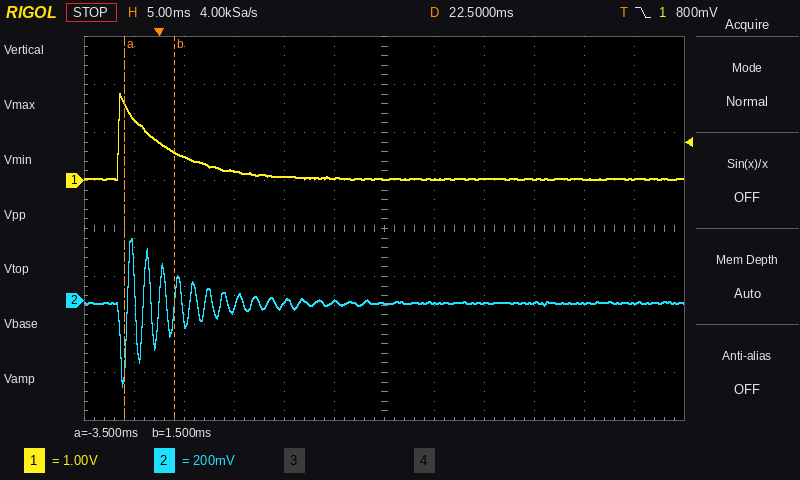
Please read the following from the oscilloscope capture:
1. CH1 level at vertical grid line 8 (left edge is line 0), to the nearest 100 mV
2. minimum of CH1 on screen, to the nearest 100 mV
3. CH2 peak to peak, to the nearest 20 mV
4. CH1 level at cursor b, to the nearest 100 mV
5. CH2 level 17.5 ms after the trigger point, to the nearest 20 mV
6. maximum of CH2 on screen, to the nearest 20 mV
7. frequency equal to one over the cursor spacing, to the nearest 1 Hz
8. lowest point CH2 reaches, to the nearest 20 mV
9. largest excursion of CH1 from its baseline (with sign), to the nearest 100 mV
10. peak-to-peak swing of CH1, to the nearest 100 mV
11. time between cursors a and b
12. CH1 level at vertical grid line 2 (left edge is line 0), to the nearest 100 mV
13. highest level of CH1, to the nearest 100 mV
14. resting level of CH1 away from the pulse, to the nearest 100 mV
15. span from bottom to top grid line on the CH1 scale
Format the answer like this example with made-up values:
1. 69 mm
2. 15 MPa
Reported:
1. 0.0 V
2. 0.0 V
3. 620 mV
4. 600 mV
5. 0 mV
6. 260 mV
7. 200 Hz
8. -360 mV
9. +1.8 V
10. 1.8 V
11. 5.0 ms
12. 500 mV
13. 1.8 V
14. 0.0 V
15. 8 V
